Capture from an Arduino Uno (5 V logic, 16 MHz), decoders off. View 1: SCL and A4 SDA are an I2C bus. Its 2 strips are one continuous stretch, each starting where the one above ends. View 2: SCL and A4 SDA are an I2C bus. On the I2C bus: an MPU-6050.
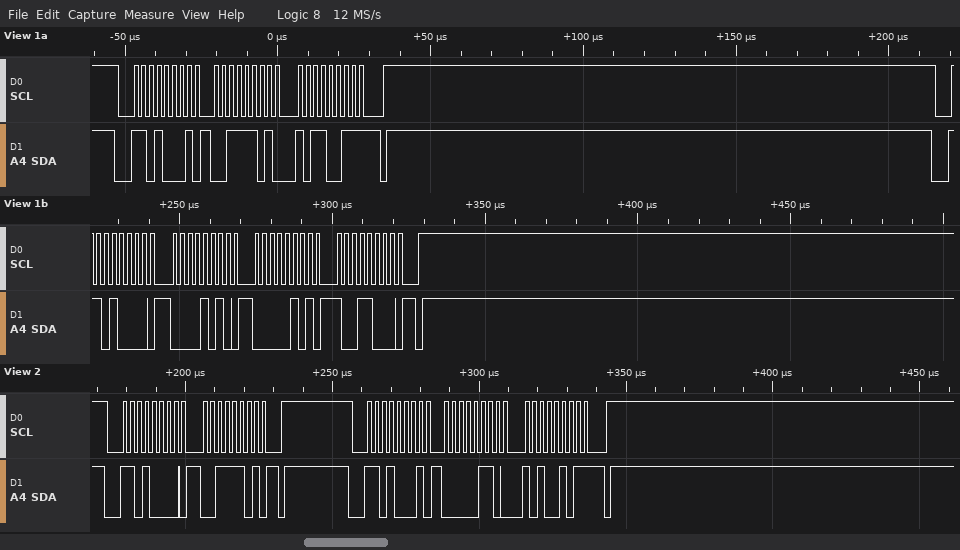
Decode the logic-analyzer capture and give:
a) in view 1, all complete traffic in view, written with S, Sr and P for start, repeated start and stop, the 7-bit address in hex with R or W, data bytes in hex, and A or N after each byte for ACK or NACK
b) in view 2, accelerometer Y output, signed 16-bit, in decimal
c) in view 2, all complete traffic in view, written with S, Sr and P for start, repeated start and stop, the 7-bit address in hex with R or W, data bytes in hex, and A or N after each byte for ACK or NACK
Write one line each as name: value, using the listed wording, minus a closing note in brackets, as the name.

in view 1, all complete traffic in view, written with S, Sr and P for start, repeated start and stop, the 7-bit address in hex with R or W, data bytes in hex, and A or N after each byte for ACK or NACK: S 68R A 3D A B3 N P S 68W A 0A A 05 A 98 A P
in view 2, accelerometer Y output, signed 16-bit, in decimal: 1701
in view 2, all complete traffic in view, written with S, Sr and P for start, repeated start and stop, the 7-bit address in hex with R or W, data bytes in hex, and A or N after each byte for ACK or NACK: S 68W A 3D A P S 68R A 06 A A5 N P
